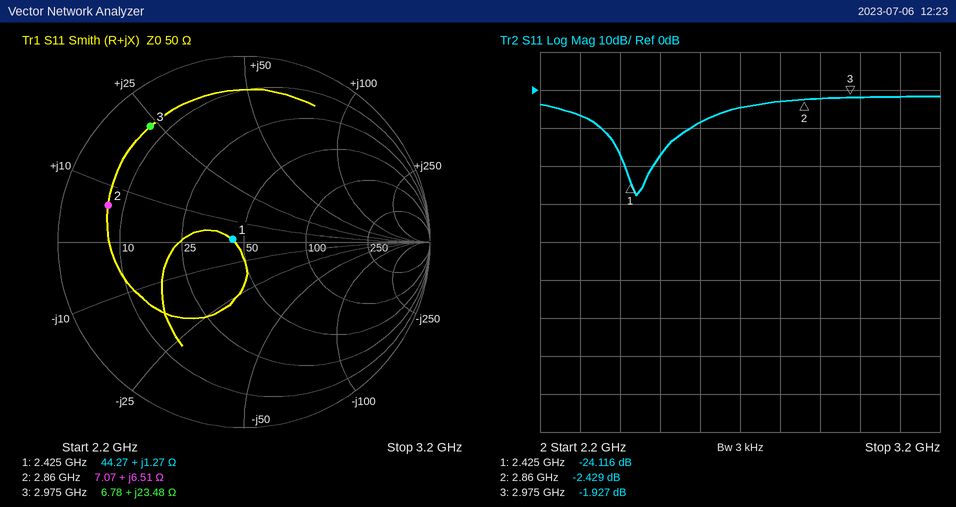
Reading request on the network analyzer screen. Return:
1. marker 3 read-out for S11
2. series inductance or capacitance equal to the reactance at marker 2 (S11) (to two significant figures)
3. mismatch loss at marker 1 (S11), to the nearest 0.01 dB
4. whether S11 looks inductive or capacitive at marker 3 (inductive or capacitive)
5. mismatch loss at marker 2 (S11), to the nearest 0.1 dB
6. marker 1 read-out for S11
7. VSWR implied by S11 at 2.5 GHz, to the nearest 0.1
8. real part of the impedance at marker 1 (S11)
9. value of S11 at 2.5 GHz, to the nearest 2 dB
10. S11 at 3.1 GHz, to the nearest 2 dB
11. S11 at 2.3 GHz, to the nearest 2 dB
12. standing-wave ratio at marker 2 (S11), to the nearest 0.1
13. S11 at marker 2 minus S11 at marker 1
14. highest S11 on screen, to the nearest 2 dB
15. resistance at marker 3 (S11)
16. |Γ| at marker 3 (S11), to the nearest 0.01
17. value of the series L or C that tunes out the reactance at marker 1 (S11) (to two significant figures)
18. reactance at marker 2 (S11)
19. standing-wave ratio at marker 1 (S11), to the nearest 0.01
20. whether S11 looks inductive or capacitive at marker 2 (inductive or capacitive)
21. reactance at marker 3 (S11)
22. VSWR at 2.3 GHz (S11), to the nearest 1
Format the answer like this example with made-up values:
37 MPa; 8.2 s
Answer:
-1.927 dB; 360 pH; 0.02 dB; inductive; 3.7 dB; -24.116 dB; 1.3; 44.27 Ω; -18 dB; -2 dB; -6 dB; 7.2; 21.687 dB; -2 dB; 6.78 Ω; 0.80; 52 pF; +6.51 Ω; 1.13; inductive; +23.48 Ω; 3
